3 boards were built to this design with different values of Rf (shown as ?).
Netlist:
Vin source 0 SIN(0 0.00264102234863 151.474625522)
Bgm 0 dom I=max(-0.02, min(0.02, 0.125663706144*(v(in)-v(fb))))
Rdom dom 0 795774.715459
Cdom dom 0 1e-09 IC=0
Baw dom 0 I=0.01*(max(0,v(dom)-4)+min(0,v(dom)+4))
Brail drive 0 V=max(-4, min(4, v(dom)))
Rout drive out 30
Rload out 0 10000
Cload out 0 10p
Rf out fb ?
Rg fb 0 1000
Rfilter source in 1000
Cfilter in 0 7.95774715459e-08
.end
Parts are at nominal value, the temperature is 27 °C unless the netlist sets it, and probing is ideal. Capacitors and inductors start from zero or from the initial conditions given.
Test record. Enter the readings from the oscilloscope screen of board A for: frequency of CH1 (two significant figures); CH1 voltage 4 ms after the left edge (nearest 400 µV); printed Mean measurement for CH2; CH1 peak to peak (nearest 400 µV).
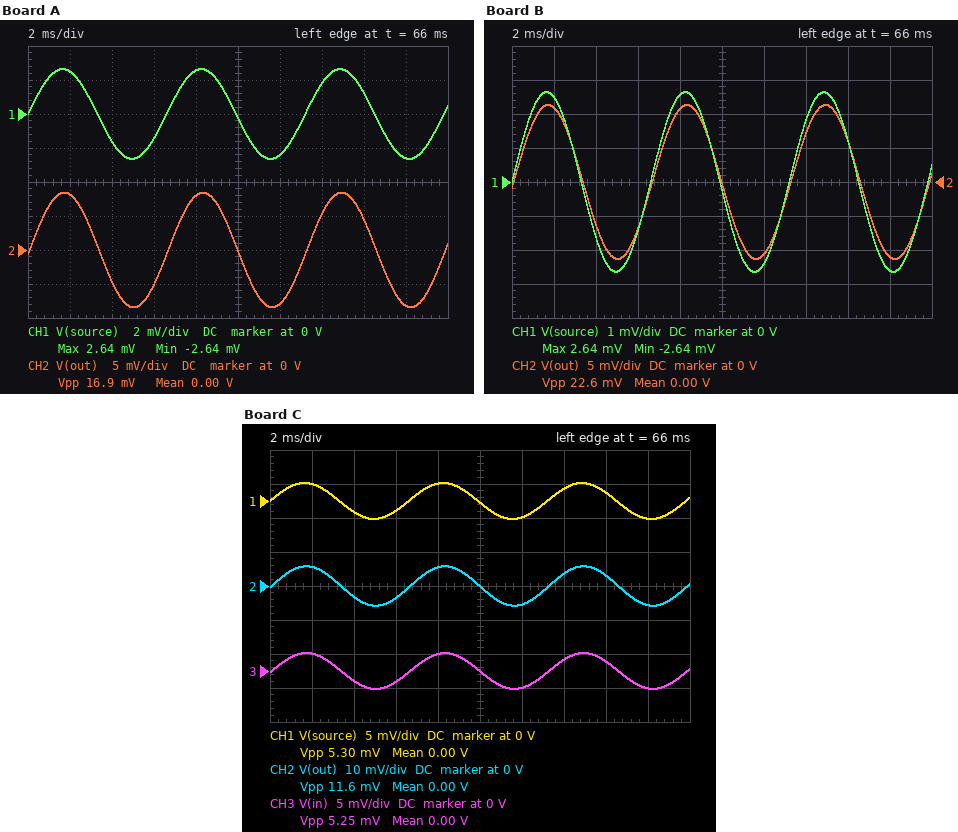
150 Hz
-1.6 mV
0.00 V
5.2 mV
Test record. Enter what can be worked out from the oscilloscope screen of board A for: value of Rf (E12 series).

2.2 kΩ
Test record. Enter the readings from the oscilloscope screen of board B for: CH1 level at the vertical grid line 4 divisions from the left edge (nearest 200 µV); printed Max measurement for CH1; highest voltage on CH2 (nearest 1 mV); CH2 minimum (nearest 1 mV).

2.6 mV
2.64 mV
11 mV
-11 mV
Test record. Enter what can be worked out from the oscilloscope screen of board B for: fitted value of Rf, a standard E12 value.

3.3 kΩ
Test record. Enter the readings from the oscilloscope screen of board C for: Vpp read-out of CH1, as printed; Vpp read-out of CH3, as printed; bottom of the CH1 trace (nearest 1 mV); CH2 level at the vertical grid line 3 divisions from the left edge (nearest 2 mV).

5.30 mV
5.25 mV
-3 mV
-4 mV
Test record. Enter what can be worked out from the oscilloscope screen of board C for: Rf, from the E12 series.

1.2 kΩ
